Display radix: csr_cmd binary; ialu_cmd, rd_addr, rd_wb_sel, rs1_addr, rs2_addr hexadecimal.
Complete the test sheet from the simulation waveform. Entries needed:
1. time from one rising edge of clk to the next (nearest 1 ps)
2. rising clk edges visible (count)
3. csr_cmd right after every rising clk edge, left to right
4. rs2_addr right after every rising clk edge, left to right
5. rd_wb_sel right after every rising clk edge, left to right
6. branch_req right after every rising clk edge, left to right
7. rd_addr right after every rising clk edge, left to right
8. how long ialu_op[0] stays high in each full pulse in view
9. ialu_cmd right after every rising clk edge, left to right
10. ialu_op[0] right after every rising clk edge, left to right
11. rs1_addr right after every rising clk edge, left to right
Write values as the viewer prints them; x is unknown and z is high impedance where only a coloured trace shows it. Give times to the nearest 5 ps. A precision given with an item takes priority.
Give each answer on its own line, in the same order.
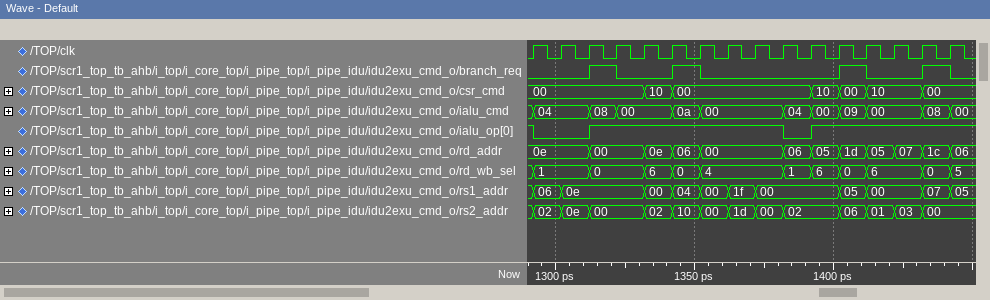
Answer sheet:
10 ps
16
00, 00, 00, 00, 10, 00, 00, 00, 00, 00, 10, 00, 10, 10, 00, 00
02, 0e, 00, 00, 02, 10, 00, 1d, 00, 02, 02, 06, 01, 03, 00, 00
1, 1, 0, 0, 6, 0, 4, 4, 4, 1, 6, 0, 6, 6, 0, 5
0 0 1 0 0 1 0 0 0 0 0 1 0 0 1 0
0e, 0e, 00, 00, 0e, 06, 00, 00, 00, 06, 05, 1d, 05, 07, 1c, 06
70 ps
04, 04, 08, 00, 00, 0a, 00, 00, 00, 04, 00, 09, 00, 00, 08, 00
0 0 1 1 1 1 1 1 1 0 1 1 1 1 1 1
06, 0e, 0e, 0e, 00, 04, 00, 1f, 00, 00, 00, 05, 00, 00, 07, 05
